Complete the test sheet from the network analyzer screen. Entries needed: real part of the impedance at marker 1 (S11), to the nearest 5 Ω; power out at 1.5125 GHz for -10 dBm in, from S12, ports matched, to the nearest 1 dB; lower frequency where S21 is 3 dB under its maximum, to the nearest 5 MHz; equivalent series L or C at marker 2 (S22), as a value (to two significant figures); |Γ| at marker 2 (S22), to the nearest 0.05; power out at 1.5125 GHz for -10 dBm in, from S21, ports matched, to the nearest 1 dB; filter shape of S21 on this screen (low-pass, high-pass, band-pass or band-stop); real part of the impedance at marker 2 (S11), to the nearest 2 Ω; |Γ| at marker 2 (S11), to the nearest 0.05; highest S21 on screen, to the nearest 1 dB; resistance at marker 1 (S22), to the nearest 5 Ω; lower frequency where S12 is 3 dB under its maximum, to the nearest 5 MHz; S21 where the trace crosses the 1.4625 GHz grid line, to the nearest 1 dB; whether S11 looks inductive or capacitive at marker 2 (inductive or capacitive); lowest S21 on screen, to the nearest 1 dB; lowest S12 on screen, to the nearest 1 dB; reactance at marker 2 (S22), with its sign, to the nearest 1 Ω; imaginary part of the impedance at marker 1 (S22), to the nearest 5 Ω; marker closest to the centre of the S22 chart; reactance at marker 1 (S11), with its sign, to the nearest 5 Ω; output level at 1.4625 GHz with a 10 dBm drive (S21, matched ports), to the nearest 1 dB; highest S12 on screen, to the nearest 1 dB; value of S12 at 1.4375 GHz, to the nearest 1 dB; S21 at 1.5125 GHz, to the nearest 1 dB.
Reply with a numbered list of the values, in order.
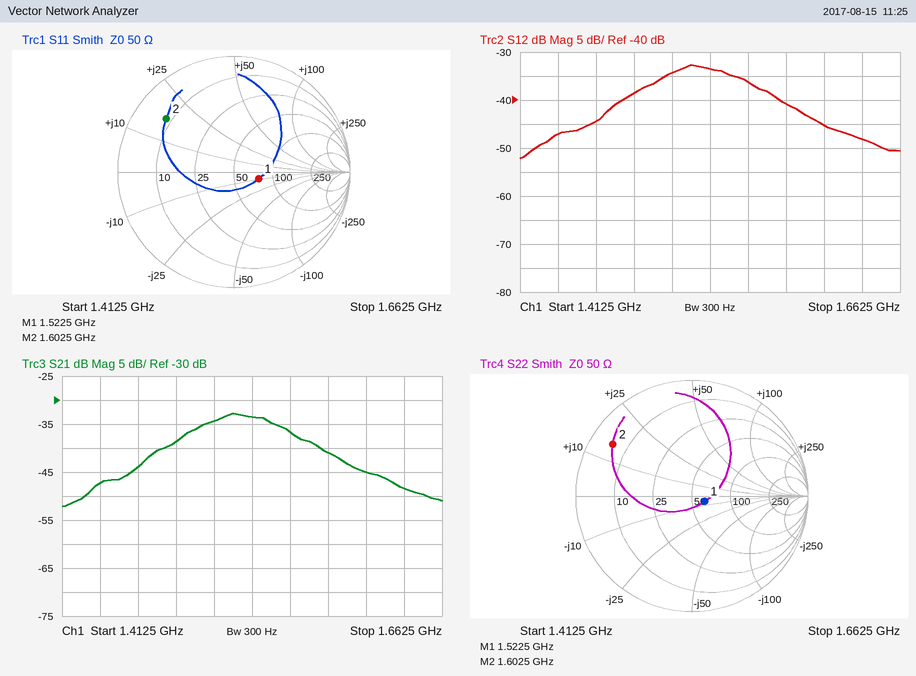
1. 75 Ω
2. -44 dBm
3. 1.500 GHz
4. 1.5 nH
5. 0.80
6. -44 dBm
7. band-pass
8. 8 Ω
9. 0.75
10. -33 dB
11. 60 Ω
12. 1.505 GHz
13. -44 dB
14. inductive
15. -52 dB
16. -52 dB
17. +15 Ω
18. -5 Ω
19. marker 1
20. -10 Ω
21. -34 dBm
22. -33 dB
23. -47 dB
24. -34 dB
